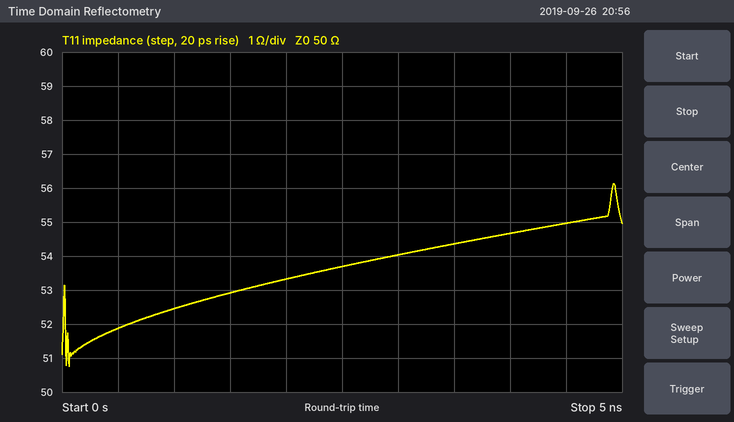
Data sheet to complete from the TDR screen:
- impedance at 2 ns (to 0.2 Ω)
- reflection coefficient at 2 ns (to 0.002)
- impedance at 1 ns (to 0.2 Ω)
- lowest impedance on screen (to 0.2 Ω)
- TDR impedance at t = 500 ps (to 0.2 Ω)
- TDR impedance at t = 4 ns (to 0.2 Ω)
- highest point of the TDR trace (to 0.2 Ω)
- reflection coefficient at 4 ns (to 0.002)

53.4 Ω
+0.032
52.4 Ω
50.8 Ω
51.8 Ω
54.6 Ω
56.2 Ω
+0.044
